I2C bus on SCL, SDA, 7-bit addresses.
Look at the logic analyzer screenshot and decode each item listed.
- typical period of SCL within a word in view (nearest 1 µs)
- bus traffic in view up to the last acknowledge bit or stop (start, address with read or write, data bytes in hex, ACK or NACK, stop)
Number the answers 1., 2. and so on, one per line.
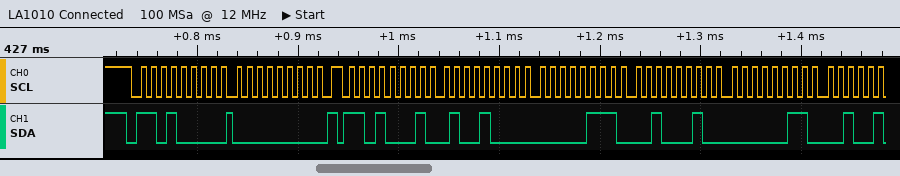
1. 10 µs
2. start, address 68 write ACK, 00 ACK, repeated start, address 68 read ACK, 48 ACK, 07 ACK, 22 ACK, 03 ACK
